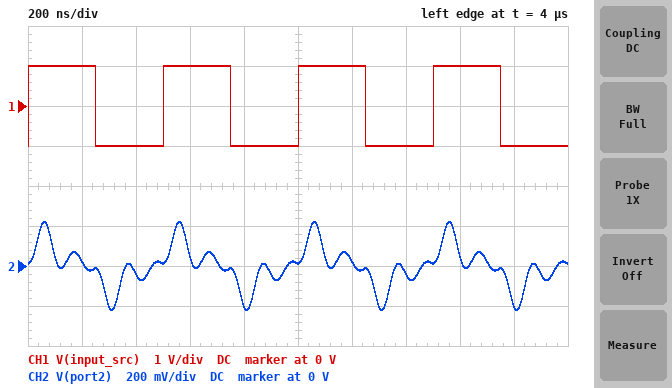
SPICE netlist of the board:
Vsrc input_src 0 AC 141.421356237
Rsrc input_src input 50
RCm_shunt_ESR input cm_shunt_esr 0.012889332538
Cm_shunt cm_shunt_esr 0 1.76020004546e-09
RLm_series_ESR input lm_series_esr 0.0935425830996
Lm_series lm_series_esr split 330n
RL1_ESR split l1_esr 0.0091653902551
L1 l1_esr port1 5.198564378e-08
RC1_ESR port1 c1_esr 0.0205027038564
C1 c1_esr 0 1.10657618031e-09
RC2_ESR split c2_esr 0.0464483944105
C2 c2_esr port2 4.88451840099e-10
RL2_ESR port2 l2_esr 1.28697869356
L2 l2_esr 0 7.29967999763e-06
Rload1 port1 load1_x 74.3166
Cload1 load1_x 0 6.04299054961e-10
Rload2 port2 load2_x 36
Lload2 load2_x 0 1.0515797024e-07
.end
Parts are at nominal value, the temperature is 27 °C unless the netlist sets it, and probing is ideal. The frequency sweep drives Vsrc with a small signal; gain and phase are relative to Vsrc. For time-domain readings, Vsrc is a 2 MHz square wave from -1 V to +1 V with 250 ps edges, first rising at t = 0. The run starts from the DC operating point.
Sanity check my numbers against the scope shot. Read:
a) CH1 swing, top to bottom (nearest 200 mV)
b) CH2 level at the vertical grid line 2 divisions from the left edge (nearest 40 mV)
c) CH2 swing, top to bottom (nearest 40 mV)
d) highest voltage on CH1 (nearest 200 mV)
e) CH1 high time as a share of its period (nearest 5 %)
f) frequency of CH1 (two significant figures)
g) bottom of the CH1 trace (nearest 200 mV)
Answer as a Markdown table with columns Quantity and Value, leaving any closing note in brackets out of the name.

| Quantity | Value |
|---|---|
| CH1 swing, top to bottom | 2.0 V |
| CH2 level at the vertical grid line 2 divisions from the left edge | -40 mV |
| CH2 swing, top to bottom | 440 mV |
| highest voltage on CH1 | 1.0 V |
| CH1 high time as a share of its period | 50 % |
| frequency of CH1 | 2.0 MHz |
| bottom of the CH1 trace | -1.0 V |
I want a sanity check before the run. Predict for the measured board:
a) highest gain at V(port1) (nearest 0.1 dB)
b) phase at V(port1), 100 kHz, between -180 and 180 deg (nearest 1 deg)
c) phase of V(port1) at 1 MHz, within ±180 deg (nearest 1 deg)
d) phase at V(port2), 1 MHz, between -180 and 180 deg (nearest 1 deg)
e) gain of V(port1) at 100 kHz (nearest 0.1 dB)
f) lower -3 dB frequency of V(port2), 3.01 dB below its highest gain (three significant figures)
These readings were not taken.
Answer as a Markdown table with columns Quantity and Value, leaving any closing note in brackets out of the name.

| Quantity | Value |
|---|---|
| highest gain at V(port1) | 0 dB |
| phase at V(port1), 100 kHz, between -180 and 180 deg | -7 deg |
| phase of V(port1) at 1 MHz, within ±180 deg | -50 deg |
| phase at V(port2), 1 MHz, between -180 and 180 deg | 74 deg |
| gain of V(port1) at 100 kHz | -0.1 dB |
| lower -3 dB frequency of V(port2), 3.01 dB below its highest gain | 7.43 MHz |
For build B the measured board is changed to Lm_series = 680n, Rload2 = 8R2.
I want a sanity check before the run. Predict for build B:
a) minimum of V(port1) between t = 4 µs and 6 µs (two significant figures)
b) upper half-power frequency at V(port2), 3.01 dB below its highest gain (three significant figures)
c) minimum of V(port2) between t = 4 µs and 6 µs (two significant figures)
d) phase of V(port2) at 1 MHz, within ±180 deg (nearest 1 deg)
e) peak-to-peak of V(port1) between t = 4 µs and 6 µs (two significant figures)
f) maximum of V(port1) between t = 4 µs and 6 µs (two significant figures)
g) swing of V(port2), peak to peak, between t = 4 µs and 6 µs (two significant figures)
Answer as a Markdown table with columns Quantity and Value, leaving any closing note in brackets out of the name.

| Quantity | Value |
|---|---|
| minimum of V(port1) between t = 4 µs and 6 µs | -690 mV |
| upper half-power frequency at V(port2), 3.01 dB below its highest gain | 7.04 MHz |
| minimum of V(port2) between t = 4 µs and 6 µs | -72 mV |
| phase of V(port2) at 1 MHz, within ±180 deg | 53 deg |
| peak-to-peak of V(port1) between t = 4 µs and 6 µs | 1.4 V |
| maximum of V(port1) between t = 4 µs and 6 µs | 690 mV |
| swing of V(port2), peak to peak, between t = 4 µs and 6 µs | 140 mV |
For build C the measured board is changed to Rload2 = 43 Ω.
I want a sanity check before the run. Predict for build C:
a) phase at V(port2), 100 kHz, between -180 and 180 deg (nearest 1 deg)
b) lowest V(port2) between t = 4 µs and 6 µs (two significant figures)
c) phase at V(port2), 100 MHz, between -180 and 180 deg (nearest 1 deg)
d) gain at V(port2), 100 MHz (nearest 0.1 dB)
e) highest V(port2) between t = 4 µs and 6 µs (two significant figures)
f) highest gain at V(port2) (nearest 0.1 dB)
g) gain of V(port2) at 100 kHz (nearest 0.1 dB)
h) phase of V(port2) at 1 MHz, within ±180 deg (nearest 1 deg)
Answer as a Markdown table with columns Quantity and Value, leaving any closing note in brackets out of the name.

| Quantity | Value |
|---|---|
| phase at V(port2), 100 kHz, between -180 and 180 deg | 151 deg |
| lowest V(port2) between t = 4 µs and 6 µs | -260 mV |
| phase at V(port2), 100 MHz, between -180 and 180 deg | -96 deg |
| gain at V(port2), 100 MHz | -54.6 dB |
| highest V(port2) between t = 4 µs and 6 µs | 260 mV |
| highest gain at V(port2) | -10.3 dB |
| gain of V(port2) at 100 kHz | -57.1 dB |
| phase of V(port2) at 1 MHz, within ±180 deg | 79 deg |
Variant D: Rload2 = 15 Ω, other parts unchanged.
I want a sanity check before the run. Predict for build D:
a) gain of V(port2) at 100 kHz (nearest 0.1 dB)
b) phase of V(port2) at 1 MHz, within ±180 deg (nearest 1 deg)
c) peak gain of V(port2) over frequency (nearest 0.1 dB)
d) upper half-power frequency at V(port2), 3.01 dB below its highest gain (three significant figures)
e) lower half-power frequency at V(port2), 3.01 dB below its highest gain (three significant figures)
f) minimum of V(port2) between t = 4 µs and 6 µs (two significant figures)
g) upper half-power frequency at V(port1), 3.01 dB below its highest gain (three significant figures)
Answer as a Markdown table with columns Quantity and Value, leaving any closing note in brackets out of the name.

| Quantity | Value |
|---|---|
| gain of V(port2) at 100 kHz | -57.8 dB |
| phase of V(port2) at 1 MHz, within ±180 deg | 58 deg |
| peak gain of V(port2) over frequency | -14.7 dB |
| upper half-power frequency at V(port2), 3.01 dB below its highest gain | 9.88 MHz |
| lower half-power frequency at V(port2), 3.01 dB below its highest gain | 7.80 MHz |
| minimum of V(port2) between t = 4 µs and 6 µs | -100 mV |
| upper half-power frequency at V(port1), 3.01 dB below its highest gain | 802 kHz |
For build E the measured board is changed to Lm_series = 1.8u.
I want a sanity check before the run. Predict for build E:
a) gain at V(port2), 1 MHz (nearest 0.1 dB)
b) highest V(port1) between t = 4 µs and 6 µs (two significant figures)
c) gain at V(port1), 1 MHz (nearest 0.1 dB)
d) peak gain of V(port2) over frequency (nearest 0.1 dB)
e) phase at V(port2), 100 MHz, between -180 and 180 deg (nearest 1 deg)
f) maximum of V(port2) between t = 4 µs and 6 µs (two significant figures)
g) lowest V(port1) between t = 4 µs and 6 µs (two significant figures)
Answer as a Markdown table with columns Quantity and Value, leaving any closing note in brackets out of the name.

| Quantity | Value |
|---|---|
| gain at V(port2), 1 MHz | -24.3 dB |
| highest V(port1) between t = 4 µs and 6 µs | 620 mV |
| gain at V(port1), 1 MHz | -3.3 dB |
| peak gain of V(port2) over frequency | -12.1 dB |
| phase at V(port2), 100 MHz, between -180 and 180 deg | -96 deg |
| maximum of V(port2) between t = 4 µs and 6 µs | 160 mV |
| lowest V(port1) between t = 4 µs and 6 µs | -620 mV |
